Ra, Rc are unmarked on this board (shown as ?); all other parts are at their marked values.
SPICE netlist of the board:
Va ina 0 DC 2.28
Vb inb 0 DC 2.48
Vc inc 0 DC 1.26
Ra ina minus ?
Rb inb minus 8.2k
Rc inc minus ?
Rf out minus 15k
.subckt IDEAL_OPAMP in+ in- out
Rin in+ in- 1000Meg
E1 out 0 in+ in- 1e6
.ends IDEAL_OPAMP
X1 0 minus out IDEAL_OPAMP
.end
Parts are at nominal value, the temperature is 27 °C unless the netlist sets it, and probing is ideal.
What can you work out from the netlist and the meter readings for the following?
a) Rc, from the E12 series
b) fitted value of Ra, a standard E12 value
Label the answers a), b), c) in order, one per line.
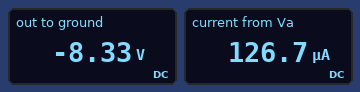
a) 10 kΩ
b) 18 kΩ
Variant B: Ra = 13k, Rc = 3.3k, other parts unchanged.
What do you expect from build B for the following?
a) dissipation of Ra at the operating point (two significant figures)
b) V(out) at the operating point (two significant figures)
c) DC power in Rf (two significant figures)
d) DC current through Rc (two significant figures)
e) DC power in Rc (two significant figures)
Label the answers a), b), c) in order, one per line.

a) 400 µW
b) -13 V
c) 11 mW
d) 380 µA
e) 480 µW
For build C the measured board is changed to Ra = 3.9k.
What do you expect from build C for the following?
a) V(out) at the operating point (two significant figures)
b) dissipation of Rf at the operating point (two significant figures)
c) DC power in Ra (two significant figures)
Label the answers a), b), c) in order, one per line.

a) -15 V
b) 15 mW
c) 1.3 mW
